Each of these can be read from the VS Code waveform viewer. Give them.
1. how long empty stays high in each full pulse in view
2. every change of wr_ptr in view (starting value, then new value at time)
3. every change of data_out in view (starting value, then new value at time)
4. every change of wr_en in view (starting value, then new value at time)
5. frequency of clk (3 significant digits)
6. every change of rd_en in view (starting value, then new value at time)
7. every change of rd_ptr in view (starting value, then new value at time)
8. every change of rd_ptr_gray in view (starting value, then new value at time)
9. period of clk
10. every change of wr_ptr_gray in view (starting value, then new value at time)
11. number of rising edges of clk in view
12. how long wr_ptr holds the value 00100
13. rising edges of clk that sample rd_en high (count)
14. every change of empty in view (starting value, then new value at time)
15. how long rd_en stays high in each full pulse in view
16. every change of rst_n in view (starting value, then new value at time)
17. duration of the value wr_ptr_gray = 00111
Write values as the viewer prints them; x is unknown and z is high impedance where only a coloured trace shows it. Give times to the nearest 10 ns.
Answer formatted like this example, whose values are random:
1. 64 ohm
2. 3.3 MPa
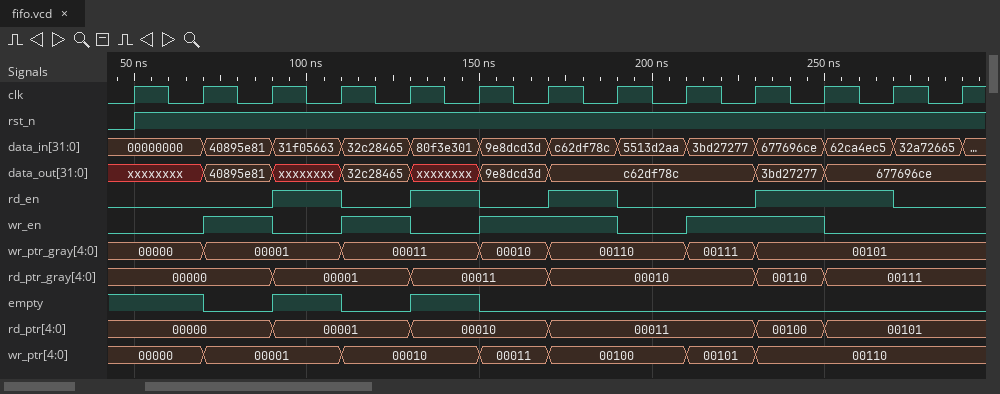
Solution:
1. 20 ns, 20 ns
2. 00000, 00001 at 70 ns, 00010 at 110 ns, 00011 at 150 ns, 00100 at 170 ns, 00101 at 210 ns, 00110 at 230 ns
3. xxxxxxxx, 40895e81 at 70 ns, xxxxxxxx at 90 ns, 32c28465 at 110 ns, xxxxxxxx at 130 ns, 9e8dcd3d at 150 ns, c62df78c at 170 ns, 3bd27277 at 230 ns, 677696ce at 250 ns
4. 0, 1 at 70 ns, 0 at 90 ns, 1 at 110 ns, 0 at 130 ns, 1 at 150 ns, 0 at 190 ns, 1 at 210 ns, 0 at 250 ns
5. 50.0 MHz
6. 0, 1 at 90 ns, 0 at 110 ns, 1 at 130 ns, 0 at 150 ns, 1 at 170 ns, 0 at 190 ns, 1 at 230 ns, 0 at 270 ns
7. 00000, 00001 at 90 ns, 00010 at 130 ns, 00011 at 170 ns, 00100 at 230 ns, 00101 at 250 ns
8. 00000, 00001 at 90 ns, 00011 at 130 ns, 00010 at 170 ns, 00110 at 230 ns, 00111 at 250 ns
9. 20 ns
10. 00000, 00001 at 70 ns, 00011 at 110 ns, 00010 at 150 ns, 00110 at 170 ns, 00111 at 210 ns, 00101 at 230 ns
11. 13
12. 40 ns
13. 5
14. 1, 0 at 70 ns, 1 at 90 ns, 0 at 110 ns, 1 at 130 ns, 0 at 150 ns
15. 20 ns, 20 ns, 20 ns, 40 ns
16. 0, 1 at 50 ns
17. 20 ns
